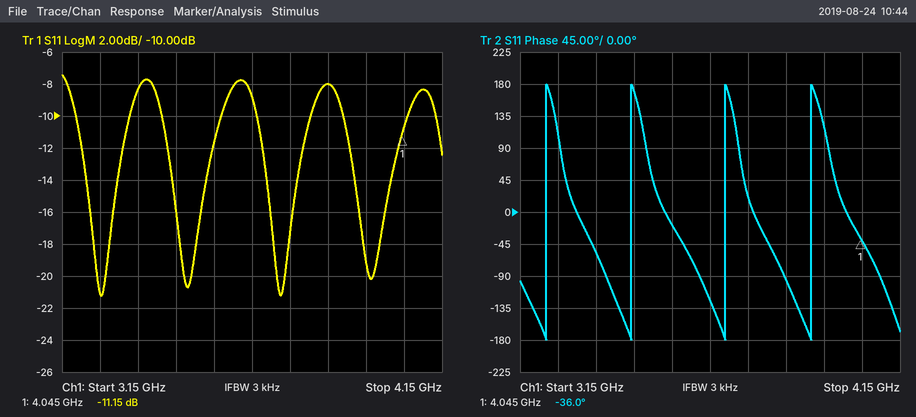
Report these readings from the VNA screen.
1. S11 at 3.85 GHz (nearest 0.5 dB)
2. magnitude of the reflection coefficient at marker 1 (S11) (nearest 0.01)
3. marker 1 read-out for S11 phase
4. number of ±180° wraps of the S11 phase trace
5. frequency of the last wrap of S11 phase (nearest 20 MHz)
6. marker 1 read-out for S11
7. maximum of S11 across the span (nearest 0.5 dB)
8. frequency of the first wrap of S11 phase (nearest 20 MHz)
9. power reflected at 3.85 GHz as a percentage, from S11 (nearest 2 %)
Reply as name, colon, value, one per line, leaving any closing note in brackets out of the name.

S11 at 3.85 GHz: -8.0 dB
magnitude of the reflection coefficient at marker 1 (S11): 0.28
marker 1 read-out for S11 phase: -36.0°
number of ±180° wraps of the S11 phase trace: 4
frequency of the last wrap of S11 phase: 3.92 GHz
marker 1 read-out for S11: -11.15 dB
maximum of S11 across the span: -7.5 dB
frequency of the first wrap of S11 phase: 3.22 GHz
power reflected at 3.85 GHz as a percentage, from S11: 16 %
